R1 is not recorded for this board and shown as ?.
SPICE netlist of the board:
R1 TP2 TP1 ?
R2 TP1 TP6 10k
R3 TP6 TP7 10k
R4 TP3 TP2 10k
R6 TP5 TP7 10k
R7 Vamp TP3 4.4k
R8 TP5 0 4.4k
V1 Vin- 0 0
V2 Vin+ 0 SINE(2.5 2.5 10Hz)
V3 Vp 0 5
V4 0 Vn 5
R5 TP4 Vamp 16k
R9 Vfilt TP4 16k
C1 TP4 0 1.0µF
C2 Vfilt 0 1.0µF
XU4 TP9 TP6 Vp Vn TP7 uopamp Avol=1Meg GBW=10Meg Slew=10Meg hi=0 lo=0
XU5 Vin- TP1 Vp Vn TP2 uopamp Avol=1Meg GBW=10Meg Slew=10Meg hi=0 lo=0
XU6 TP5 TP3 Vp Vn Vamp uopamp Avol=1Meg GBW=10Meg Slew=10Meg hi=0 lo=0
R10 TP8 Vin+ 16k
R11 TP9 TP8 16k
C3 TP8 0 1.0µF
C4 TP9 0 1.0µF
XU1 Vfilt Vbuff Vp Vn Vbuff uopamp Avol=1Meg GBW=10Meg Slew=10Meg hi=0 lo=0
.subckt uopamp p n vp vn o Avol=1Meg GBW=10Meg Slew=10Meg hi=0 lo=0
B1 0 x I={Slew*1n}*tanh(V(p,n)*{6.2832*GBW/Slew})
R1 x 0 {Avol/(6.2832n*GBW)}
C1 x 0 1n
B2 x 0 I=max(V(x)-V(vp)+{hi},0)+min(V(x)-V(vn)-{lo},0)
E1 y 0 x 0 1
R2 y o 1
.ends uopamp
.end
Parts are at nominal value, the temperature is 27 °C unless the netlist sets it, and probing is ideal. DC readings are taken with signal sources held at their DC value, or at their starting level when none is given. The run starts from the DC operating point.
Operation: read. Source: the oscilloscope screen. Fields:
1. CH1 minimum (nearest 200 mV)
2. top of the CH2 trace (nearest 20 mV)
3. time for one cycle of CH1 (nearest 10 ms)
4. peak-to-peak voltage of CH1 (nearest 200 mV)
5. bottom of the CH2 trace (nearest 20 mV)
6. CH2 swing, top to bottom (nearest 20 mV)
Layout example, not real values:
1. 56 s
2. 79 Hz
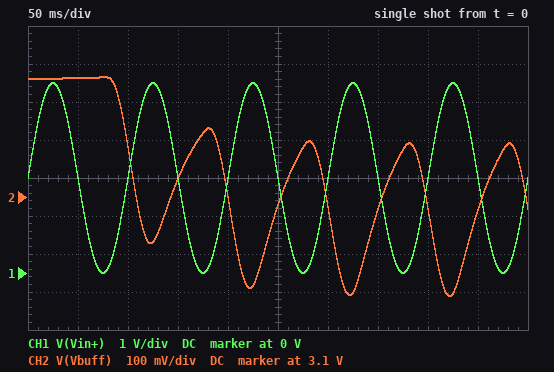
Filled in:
1. 0 V
2. 3.42 V
3. 100 ms
4. 5.0 V
5. 2.84 V
6. 580 mV
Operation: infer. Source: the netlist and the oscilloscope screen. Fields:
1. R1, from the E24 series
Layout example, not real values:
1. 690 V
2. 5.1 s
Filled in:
1. 11 kΩ
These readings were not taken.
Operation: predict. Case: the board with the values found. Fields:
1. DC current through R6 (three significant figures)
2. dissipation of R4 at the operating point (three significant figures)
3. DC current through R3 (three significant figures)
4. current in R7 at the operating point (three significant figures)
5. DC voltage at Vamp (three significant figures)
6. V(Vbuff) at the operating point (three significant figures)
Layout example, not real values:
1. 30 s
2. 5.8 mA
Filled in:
1. 347 µA
2. 1.83 mW
3. 250 µA
4. 428 µA
5. 3.41 V
6. 3.41 V
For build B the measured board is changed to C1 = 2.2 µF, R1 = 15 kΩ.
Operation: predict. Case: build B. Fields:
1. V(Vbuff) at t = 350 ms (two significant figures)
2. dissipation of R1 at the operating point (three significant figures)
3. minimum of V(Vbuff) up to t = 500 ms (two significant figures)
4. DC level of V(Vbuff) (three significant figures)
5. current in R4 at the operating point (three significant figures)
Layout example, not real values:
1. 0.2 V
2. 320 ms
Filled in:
1. 3.4 V
2. 937 µW
3. 3.3 V
4. 3.85 V
5. 528 µA
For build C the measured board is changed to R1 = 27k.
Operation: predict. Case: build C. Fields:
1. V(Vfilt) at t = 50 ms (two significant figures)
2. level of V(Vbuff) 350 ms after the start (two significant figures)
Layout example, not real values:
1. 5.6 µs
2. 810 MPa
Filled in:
1. 4.3 V
2. 4.1 V
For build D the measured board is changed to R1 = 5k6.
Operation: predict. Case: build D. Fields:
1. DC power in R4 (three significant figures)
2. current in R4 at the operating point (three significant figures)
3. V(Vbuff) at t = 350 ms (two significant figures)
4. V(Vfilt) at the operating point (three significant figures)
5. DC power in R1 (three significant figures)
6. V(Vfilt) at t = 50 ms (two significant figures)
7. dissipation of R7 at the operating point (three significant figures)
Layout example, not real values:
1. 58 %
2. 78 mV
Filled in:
1. 857 µW
2. 293 µA
3. 2.5 V
4. 2.82 V
5. 350 µW
6. 2.8 V
7. 377 µW
